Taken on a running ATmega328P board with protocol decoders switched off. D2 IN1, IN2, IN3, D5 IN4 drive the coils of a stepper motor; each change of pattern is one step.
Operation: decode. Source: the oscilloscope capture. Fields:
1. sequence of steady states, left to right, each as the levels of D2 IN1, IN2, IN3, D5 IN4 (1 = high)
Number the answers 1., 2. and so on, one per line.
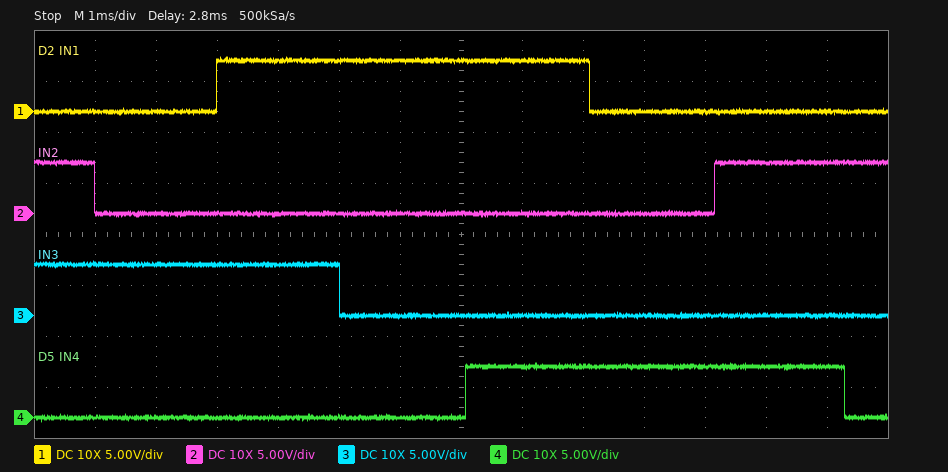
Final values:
1. 0110 0010 1010 1000 1001 0001 0101 0100
